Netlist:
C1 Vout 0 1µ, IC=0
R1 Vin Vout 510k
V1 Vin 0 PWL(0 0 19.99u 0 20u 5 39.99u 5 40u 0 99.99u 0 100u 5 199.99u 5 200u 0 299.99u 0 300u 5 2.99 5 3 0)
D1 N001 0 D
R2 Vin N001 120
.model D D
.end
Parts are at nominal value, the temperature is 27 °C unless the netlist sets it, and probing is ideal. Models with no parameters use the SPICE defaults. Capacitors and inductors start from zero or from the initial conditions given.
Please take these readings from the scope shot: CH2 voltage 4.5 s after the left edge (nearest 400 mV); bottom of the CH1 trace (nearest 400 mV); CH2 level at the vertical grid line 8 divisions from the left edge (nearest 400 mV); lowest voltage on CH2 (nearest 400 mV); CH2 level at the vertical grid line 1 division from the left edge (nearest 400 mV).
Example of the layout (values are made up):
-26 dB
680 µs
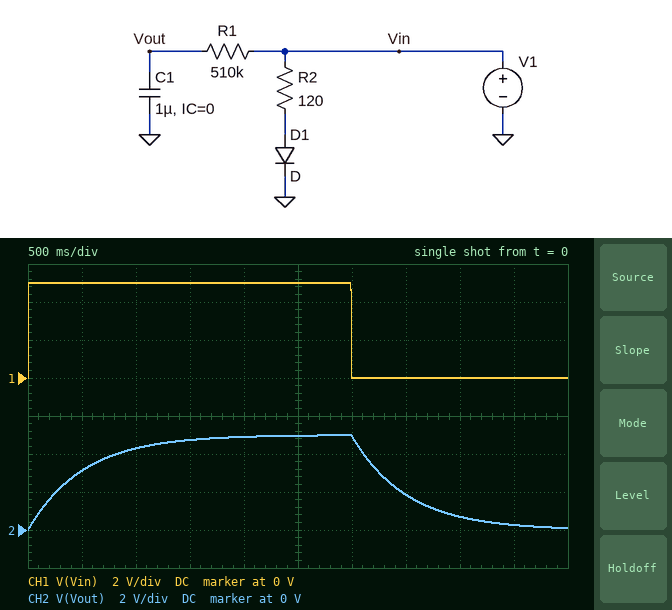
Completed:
400 mV
0 V
800 mV
0 V
3.2 V
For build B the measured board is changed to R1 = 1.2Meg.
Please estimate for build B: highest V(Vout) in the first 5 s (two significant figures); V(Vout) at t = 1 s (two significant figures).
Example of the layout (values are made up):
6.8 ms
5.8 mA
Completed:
4.6 V
2.8 V
